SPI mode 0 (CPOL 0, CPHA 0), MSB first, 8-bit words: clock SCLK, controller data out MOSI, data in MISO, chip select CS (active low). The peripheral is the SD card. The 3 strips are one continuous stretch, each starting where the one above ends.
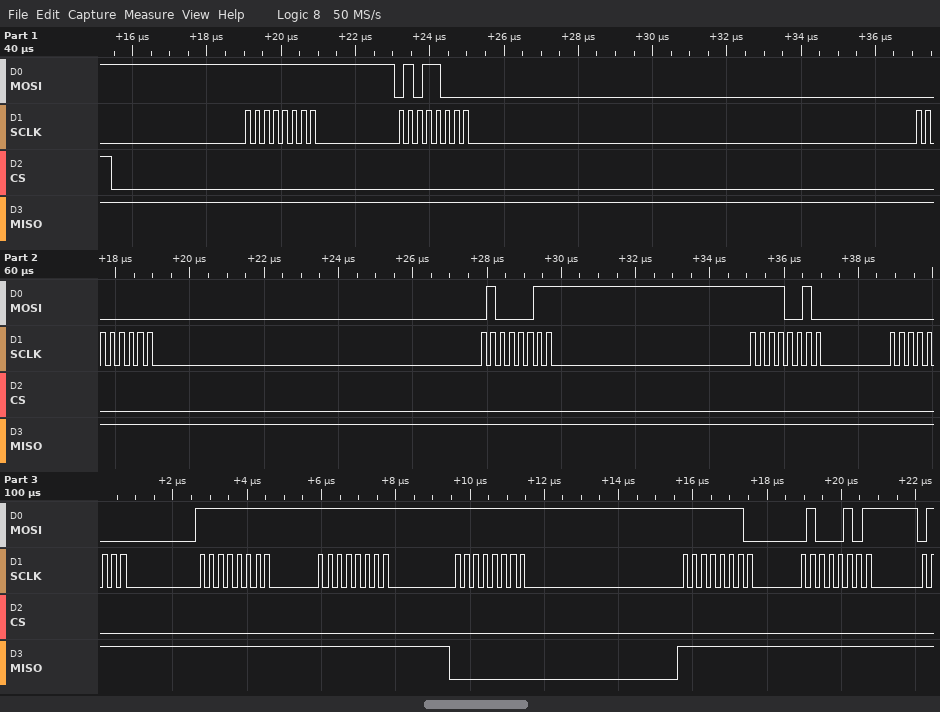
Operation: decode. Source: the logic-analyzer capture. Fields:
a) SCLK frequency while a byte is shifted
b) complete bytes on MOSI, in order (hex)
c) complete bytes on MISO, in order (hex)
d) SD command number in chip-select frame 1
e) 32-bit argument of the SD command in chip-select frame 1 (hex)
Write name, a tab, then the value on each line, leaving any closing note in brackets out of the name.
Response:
SCLK frequency while a byte is shifted	4 MHz
complete bytes on MOSI, in order	FF 58 00 43 F2 00 FF FF FF FE 45
complete bytes on MISO, in order	FF FF FF FF FF FF FF FF 00 FF FF
SD command number in chip-select frame 1	CMD24
32-bit argument of the SD command in chip-select frame 1	0x0043F200
